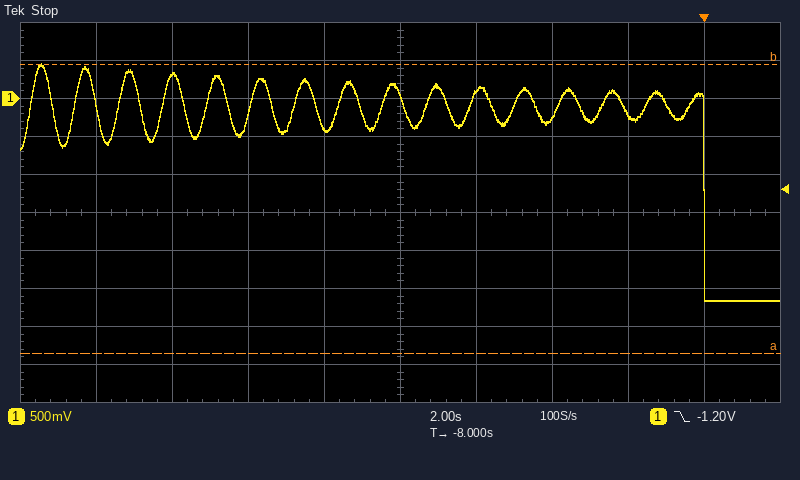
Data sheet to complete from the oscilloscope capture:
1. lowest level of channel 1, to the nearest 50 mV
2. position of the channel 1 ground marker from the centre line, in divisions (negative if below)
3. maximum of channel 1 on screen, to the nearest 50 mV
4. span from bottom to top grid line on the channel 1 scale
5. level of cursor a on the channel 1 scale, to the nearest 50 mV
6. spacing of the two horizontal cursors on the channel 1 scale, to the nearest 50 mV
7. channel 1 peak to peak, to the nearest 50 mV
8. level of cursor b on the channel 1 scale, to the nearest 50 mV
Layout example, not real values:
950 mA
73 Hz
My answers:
-2.65 V
+3.0 div
450 mV
5 V
-3.35 V
3.80 V
3.10 V
450 mV
